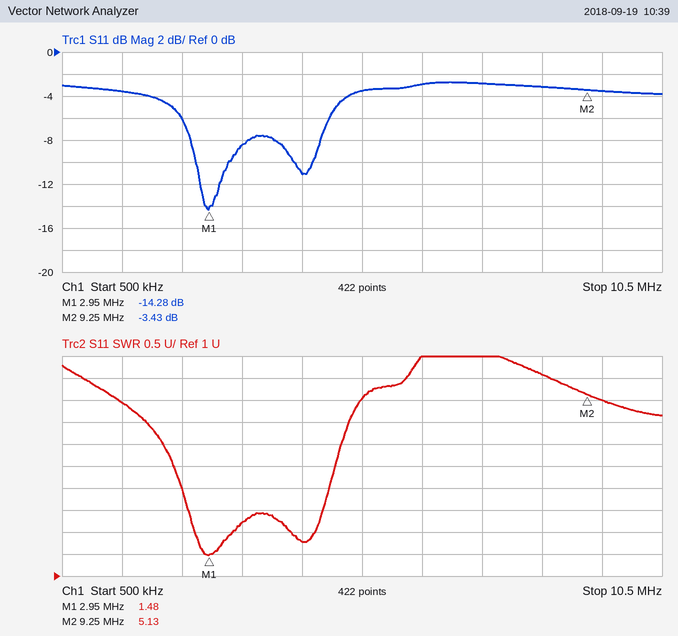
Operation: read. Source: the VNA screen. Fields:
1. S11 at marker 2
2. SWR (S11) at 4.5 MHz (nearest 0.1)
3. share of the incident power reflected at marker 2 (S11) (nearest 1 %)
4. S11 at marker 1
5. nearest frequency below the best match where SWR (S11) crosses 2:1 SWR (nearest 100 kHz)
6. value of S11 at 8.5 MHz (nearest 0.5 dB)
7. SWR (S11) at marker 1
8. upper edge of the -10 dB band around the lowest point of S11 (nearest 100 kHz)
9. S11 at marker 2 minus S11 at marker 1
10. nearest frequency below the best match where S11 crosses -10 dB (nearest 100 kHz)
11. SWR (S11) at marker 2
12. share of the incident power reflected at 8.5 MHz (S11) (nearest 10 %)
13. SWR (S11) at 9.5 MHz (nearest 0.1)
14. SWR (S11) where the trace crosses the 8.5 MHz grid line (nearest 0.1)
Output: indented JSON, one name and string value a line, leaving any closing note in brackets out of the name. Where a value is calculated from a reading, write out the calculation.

{
  "S11 at marker 2": "-3.43 dB",
  "SWR (S11) at 4.5 MHz": "1.8",
  "share of the incident power reflected at marker 2 (S11)": "10^(-3.43/10) ≈ 45 %",
  "S11 at marker 1": "-14.28 dB",
  "nearest frequency below the best match where SWR (S11) crosses 2:1 SWR": "2.7 MHz",
  "value of S11 at 8.5 MHz": "-3.0 dB",
  "SWR (S11) at marker 1": "1.48",
  "upper edge of the -10 dB band around the lowest point of S11": "3.3 MHz",
  "S11 at marker 2 minus S11 at marker 1": "-3.43 − (-14.28) = 10.85 dB",
  "nearest frequency below the best match where S11 crosses -10 dB": "2.7 MHz",
  "SWR (S11) at marker 2": "5.13",
  "share of the incident power reflected at 8.5 MHz (S11)": "10^(-3/10) ≈ 50 %",
  "SWR (S11) at 9.5 MHz": "5.0",
  "SWR (S11) where the trace crosses the 8.5 MHz grid line": "5.6"
}
